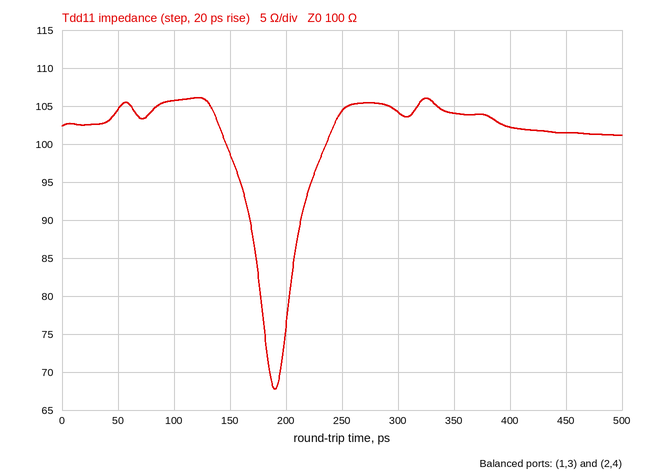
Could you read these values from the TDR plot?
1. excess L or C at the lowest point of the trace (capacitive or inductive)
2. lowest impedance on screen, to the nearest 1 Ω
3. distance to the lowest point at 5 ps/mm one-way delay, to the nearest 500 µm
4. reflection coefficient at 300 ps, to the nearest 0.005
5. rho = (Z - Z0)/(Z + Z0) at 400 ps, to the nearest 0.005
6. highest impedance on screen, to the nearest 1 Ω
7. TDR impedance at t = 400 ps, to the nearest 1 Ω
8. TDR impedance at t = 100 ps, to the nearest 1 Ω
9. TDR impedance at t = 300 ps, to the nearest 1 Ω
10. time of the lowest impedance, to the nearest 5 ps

capacitive
68 Ω
19.0 mm
+0.020
+0.010
106 Ω
102 Ω
106 Ω
104 Ω
190 ps
